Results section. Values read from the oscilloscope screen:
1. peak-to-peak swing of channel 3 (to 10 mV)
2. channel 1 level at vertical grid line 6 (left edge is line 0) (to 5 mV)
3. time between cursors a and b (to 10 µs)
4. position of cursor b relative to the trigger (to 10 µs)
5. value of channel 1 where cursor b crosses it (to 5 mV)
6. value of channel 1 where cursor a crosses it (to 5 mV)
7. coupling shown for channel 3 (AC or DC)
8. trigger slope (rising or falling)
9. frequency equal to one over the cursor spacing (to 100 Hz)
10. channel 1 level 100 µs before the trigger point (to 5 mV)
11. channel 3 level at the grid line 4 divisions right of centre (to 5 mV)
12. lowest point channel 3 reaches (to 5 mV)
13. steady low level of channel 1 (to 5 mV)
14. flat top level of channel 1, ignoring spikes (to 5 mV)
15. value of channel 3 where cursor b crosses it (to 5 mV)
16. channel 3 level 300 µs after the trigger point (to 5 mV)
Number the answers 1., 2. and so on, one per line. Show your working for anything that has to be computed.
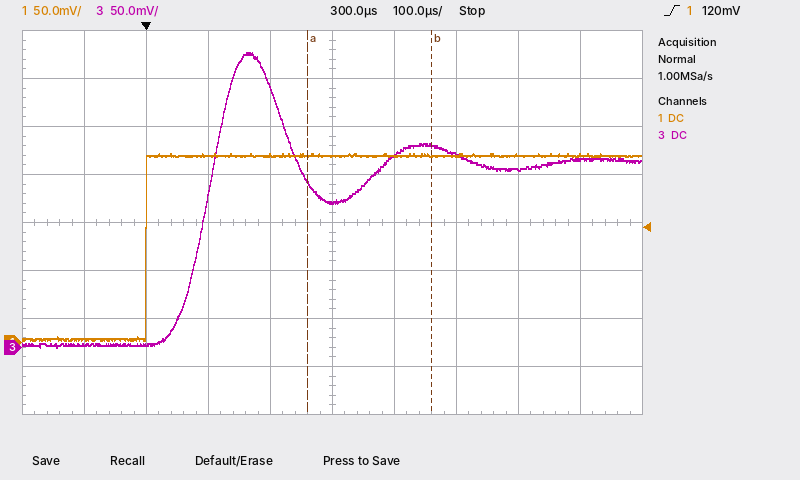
1. 310 mV
2. 195 mV
3. 200 µs
4. +460 µs
5. 195 mV
6. 195 mV
7. DC
8. rising
9. 1 / 200 µs ≈ 5.0 kHz
10. 5 mV
11. 195 mV
12. 0 mV
13. 5 mV
14. 195 mV
15. 210 mV
16. 150 mV
